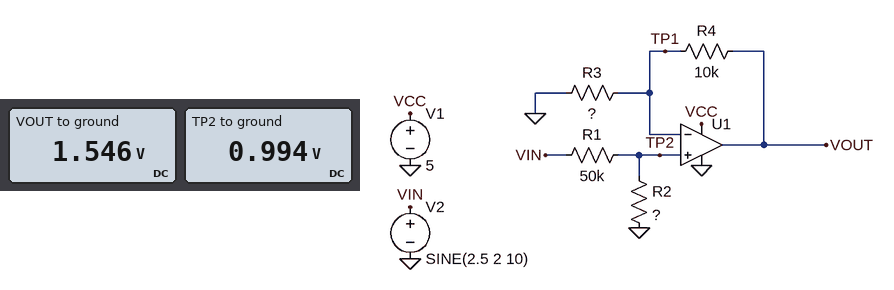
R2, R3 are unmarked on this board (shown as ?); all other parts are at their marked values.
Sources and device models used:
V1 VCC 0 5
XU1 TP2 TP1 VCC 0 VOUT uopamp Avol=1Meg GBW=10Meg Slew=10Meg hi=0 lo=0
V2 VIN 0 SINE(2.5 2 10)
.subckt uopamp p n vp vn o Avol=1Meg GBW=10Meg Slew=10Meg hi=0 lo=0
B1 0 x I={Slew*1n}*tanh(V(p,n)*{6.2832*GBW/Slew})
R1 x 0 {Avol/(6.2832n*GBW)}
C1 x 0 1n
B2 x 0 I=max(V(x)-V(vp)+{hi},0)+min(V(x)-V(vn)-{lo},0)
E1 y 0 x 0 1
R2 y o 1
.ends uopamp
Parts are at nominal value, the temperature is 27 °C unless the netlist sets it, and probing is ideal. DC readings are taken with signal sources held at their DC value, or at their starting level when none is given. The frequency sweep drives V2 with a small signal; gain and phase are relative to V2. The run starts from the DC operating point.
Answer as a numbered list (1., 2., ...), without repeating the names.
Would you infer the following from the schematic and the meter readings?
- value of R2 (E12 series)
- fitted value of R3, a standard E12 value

1. 33 kΩ
2. 18 kΩ
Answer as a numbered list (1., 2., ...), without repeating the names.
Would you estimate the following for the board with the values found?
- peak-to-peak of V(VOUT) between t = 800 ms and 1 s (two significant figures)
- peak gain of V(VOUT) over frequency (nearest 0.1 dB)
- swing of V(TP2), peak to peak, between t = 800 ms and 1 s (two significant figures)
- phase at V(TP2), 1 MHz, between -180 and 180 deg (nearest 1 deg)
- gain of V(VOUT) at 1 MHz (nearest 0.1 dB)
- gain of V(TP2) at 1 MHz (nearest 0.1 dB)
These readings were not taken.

1. 2.5 V
2. -4.2 dB
3. 1.6 V
4. 0 deg
5. -4.3 dB
6. -8.0 dB
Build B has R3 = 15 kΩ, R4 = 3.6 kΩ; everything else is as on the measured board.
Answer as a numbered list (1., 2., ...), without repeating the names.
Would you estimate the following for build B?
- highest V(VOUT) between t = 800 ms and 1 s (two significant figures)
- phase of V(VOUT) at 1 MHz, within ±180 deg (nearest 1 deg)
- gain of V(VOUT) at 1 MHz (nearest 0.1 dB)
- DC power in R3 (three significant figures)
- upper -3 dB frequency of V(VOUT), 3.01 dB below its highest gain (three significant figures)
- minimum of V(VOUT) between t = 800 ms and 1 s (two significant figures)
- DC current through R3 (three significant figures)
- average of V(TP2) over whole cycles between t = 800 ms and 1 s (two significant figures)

1. 2.2 V
2. -7 deg
3. -6.2 dB
4. 65.9 µW
5. 8.06 MHz
6. 250 mV
7. 66.3 µA
8. 990 mV
